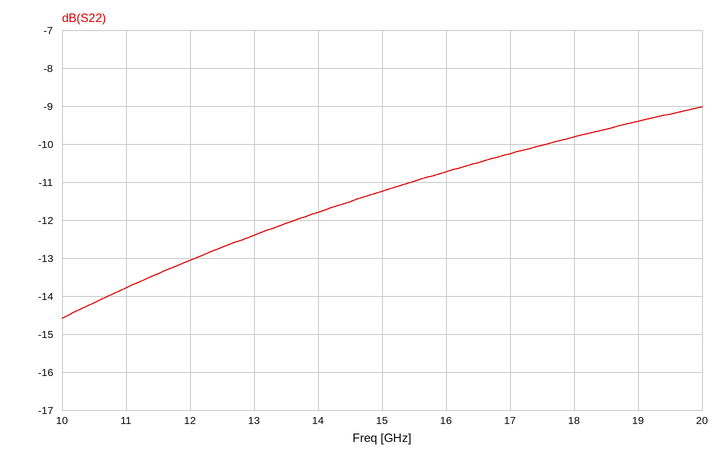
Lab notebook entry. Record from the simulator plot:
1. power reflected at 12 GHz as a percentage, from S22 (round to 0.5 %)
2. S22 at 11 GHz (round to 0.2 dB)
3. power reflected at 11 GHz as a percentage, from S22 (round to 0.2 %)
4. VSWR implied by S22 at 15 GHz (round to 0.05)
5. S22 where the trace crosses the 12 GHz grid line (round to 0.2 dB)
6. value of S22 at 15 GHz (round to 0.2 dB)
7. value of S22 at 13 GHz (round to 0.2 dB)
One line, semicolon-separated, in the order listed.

5.0 %; -13.8 dB; 4.2 %; 1.75; -13.0 dB; -11.2 dB; -12.4 dB
